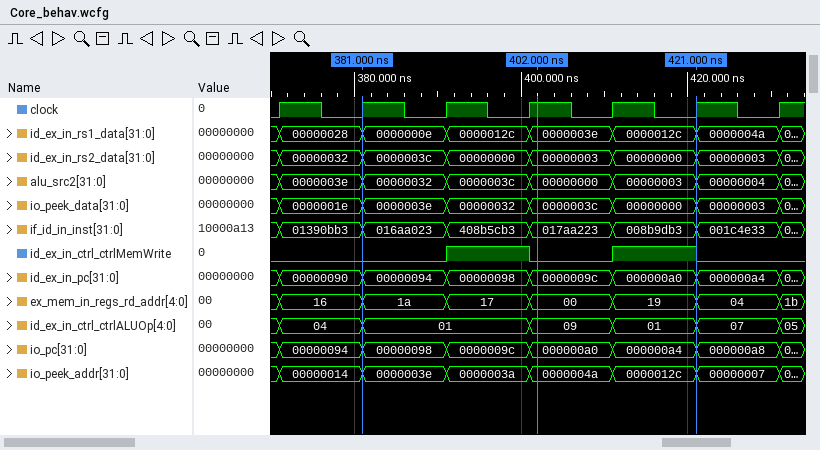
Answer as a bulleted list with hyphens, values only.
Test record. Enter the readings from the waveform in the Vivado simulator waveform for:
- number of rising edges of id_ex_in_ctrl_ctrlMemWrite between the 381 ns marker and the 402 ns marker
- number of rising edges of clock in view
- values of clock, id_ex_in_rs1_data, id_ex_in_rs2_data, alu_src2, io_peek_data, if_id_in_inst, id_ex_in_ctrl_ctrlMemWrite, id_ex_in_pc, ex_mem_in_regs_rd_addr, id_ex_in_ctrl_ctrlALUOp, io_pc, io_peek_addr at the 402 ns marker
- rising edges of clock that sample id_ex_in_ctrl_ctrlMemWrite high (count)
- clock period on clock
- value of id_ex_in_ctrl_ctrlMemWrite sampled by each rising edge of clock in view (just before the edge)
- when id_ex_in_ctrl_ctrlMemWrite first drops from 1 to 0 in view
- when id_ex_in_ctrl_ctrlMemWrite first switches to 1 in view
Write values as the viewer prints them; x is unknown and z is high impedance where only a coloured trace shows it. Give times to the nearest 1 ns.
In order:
- 1
- 7
- clock=1, id_ex_in_rs1_data=0000003e, id_ex_in_rs2_data=00000003, alu_src2=00000000, io_peek_data=0000003c, if_id_in_inst=017aa223, id_ex_in_ctrl_ctrlMemWrite=0, id_ex_in_pc=0000009c, ex_mem_in_regs_rd_addr=00, id_ex_in_ctrl_ctrlALUOp=09, io_pc=000000a0, io_peek_addr=0000004a
- 2
- 10 ns
- 0 0 0 1 0 1 0
- 401 ns
- 391 ns
